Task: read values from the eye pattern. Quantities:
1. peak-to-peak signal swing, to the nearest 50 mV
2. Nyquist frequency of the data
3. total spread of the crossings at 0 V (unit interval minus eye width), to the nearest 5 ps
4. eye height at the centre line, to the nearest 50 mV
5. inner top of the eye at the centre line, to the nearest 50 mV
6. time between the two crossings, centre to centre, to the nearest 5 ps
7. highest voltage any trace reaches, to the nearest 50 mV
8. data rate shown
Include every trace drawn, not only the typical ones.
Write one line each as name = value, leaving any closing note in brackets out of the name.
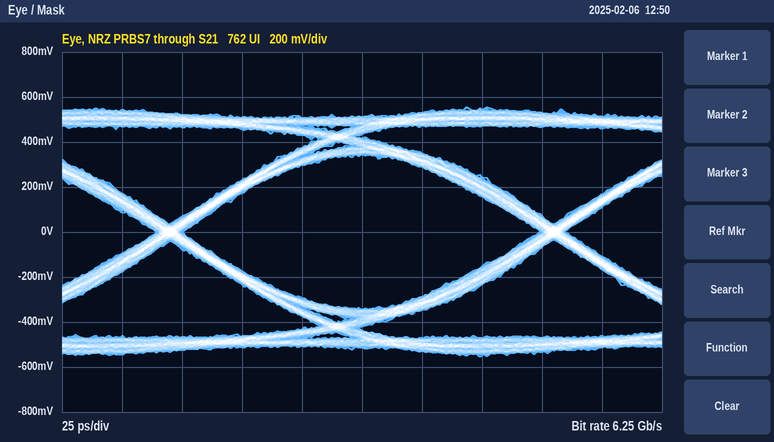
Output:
peak-to-peak signal swing, to the nearest 50 mV = 1.10 V
Nyquist frequency of the data = 3.125 GHz
total spread of the crossings at 0 V (unit interval minus eye width), to the nearest 5 ps = 10 ps
eye height at the centre line, to the nearest 50 mV = 700 mV
inner top of the eye at the centre line, to the nearest 50 mV = 350 mV
time between the two crossings, centre to centre, to the nearest 5 ps = 160 ps
highest voltage any trace reaches, to the nearest 50 mV = 550 mV
data rate shown = 6.25 Gb/s
